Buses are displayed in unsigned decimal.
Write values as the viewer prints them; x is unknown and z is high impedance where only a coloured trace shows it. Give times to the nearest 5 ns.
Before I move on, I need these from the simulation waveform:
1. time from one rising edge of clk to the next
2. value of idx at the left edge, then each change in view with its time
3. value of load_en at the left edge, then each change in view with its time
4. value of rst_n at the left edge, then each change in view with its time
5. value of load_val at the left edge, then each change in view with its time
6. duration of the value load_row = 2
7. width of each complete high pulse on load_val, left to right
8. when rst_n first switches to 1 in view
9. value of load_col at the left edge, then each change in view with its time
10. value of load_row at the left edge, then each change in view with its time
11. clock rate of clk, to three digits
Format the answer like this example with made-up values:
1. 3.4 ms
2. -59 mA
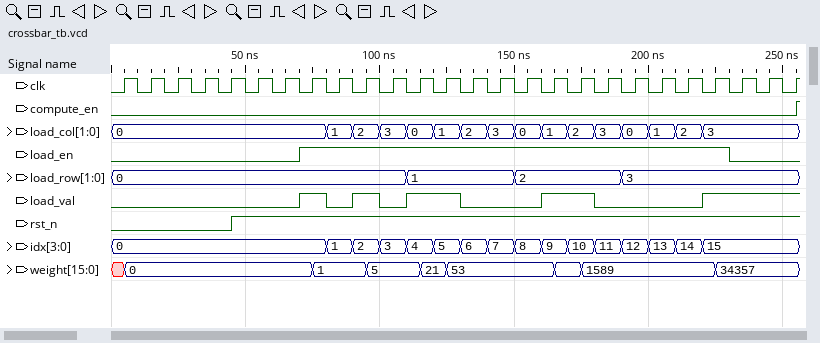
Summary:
1. 10 ns
2. 0, 1 at 80 ns, 2 at 90 ns, 3 at 100 ns, 4 at 110 ns, 5 at 120 ns, 6 at 130 ns, 7 at 140 ns, 8 at 150 ns, 9 at 160 ns, 10 at 170 ns, 11 at 180 ns, 12 at 190 ns, 13 at 200 ns, 14 at 210 ns, 15 at 220 ns
3. 0, 1 at 70 ns, 0 at 230 ns
4. 0, 1 at 45 ns
5. 0, 1 at 70 ns, 0 at 80 ns, 1 at 90 ns, 0 at 100 ns, 1 at 110 ns, 0 at 130 ns, 1 at 160 ns, 0 at 180 ns, 1 at 220 ns
6. 40 ns
7. 10 ns, 10 ns, 20 ns, 20 ns
8. 45 ns
9. 0, 1 at 80 ns, 2 at 90 ns, 3 at 100 ns, 0 at 110 ns, 1 at 120 ns, 2 at 130 ns, 3 at 140 ns, 0 at 150 ns, 1 at 160 ns, 2 at 170 ns, 3 at 180 ns, 0 at 190 ns, 1 at 200 ns, 2 at 210 ns, 3 at 220 ns
10. 0, 1 at 110 ns, 2 at 150 ns, 3 at 190 ns
11. 100 MHz
